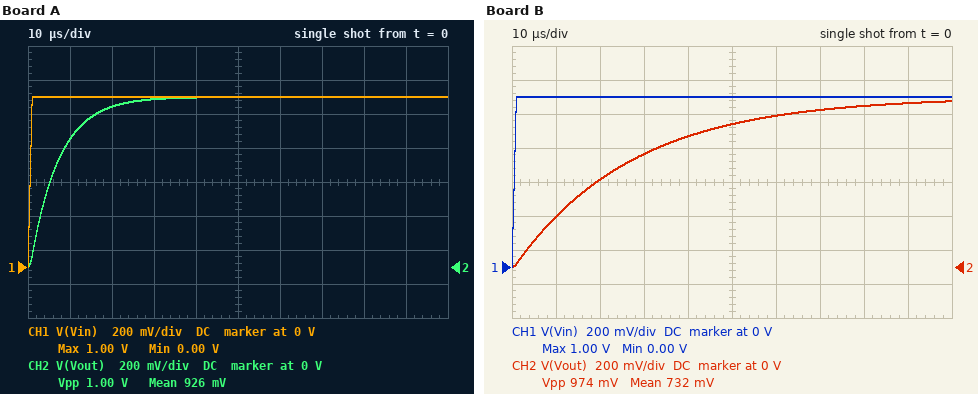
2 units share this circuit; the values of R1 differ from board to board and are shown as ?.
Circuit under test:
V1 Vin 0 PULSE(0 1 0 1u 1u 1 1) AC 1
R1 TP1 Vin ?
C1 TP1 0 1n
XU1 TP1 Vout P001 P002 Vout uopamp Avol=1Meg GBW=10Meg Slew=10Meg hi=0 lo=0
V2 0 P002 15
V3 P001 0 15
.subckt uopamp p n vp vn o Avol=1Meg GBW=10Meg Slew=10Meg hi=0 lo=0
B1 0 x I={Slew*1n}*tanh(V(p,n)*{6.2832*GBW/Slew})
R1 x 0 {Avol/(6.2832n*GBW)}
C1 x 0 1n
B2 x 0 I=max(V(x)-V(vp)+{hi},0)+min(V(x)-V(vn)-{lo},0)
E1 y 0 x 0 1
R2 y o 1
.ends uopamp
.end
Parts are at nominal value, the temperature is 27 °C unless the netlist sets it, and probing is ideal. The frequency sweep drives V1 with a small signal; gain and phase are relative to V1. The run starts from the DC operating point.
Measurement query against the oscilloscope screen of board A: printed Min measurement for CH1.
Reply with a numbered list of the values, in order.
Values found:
1. 0.00 V
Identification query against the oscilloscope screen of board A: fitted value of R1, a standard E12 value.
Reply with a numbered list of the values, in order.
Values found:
1. 6.8 kΩ
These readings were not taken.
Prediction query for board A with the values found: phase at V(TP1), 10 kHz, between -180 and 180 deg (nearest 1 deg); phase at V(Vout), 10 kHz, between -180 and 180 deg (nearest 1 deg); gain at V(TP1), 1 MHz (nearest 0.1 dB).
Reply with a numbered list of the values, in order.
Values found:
1. -23 deg
2. -23 deg
3. -32.6 dB
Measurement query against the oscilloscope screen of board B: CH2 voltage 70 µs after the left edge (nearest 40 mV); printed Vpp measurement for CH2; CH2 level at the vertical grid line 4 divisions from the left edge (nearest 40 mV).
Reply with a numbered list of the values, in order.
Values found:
1. 920 mV
2. 974 mV
3. 760 mV
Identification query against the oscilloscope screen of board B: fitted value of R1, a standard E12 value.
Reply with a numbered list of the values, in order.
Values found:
1. 27 kΩ
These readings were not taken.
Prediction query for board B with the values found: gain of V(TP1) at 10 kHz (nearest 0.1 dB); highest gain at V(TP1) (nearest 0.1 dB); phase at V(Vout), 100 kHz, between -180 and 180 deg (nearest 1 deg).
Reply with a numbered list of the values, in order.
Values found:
1. -5.9 dB
2. 0 dB
3. -87 deg
